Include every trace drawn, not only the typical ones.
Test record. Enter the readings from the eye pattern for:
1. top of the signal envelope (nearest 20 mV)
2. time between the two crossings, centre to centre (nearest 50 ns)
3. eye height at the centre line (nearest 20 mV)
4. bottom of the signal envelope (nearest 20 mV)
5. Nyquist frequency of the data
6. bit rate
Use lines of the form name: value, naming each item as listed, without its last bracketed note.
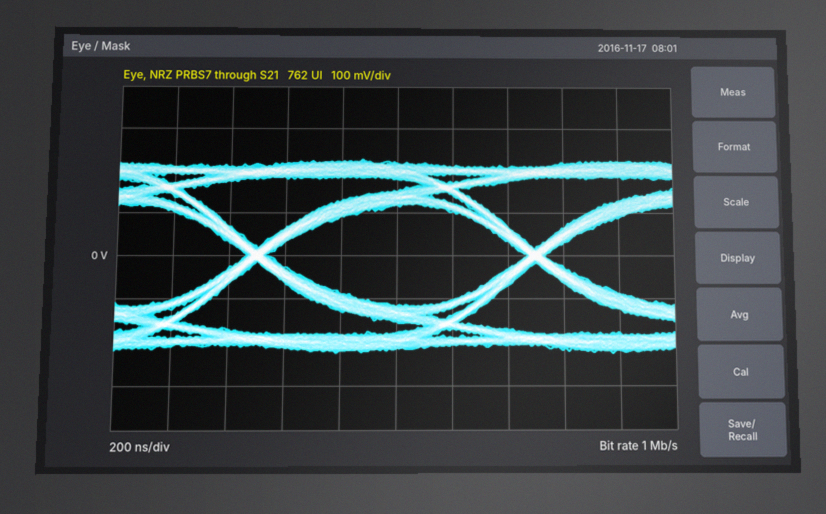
top of the signal envelope: 220 mV
time between the two crossings, centre to centre: 1.00 µs
eye height at the centre line: 240 mV
bottom of the signal envelope: -220 mV
Nyquist frequency of the data: 500 kHz
bit rate: 1 Mb/s
